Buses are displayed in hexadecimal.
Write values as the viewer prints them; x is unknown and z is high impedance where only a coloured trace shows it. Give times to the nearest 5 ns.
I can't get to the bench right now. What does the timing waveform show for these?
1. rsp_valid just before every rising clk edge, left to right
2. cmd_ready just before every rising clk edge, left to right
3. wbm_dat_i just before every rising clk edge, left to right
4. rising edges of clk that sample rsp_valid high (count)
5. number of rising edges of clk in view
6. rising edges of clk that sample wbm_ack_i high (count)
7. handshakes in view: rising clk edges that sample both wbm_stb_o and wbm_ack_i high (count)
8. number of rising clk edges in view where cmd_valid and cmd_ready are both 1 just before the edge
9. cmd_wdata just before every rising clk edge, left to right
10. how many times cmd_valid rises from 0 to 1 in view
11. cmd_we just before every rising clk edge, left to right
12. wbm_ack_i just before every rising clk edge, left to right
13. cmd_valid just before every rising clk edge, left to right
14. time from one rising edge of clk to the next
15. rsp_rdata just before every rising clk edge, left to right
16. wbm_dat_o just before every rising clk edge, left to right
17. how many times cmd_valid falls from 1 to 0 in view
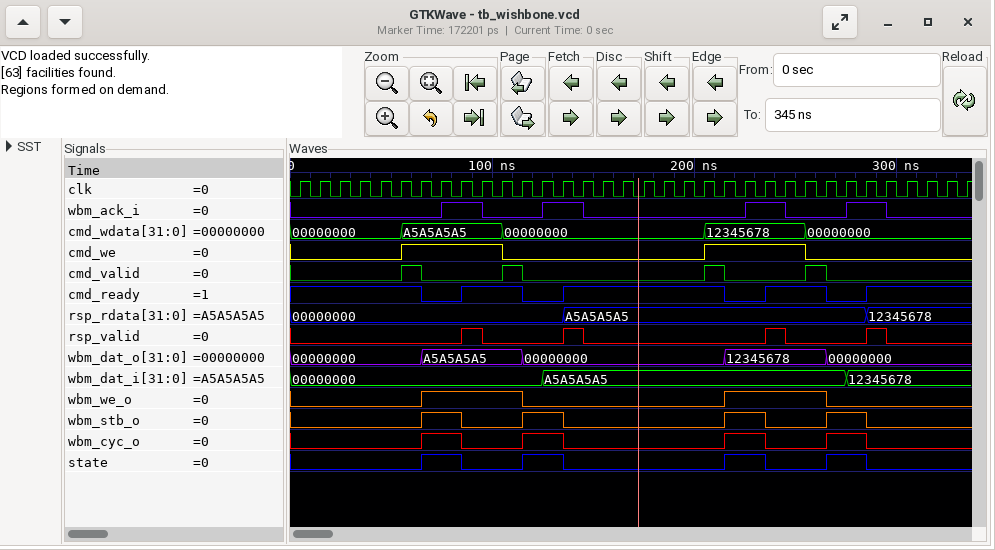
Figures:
0 0 0 0 0 0 0 0 0 1 0 0 0 0 1 0 0 0 0 0 0 0 0 0 1 0 0 0 0 1 0 0 0 0
1 1 1 1 1 1 1 0 0 1 1 1 0 0 1 1 1 1 1 1 1 1 0 0 1 1 1 0 0 1 1 1 1 1
00000000, 00000000, 00000000, 00000000, 00000000, 00000000, 00000000, 00000000, 00000000, 00000000, 00000000, 00000000, 00000000, A5A5A5A5, A5A5A5A5, A5A5A5A5, A5A5A5A5, A5A5A5A5, A5A5A5A5, A5A5A5A5, A5A5A5A5, A5A5A5A5, A5A5A5A5, A5A5A5A5, A5A5A5A5, A5A5A5A5, A5A5A5A5, A5A5A5A5, 12345678, 12345678, 12345678, 12345678, 12345678, 12345678
4
34
8
4
4
00000000, 00000000, 00000000, 00000000, 00000000, 00000000, A5A5A5A5, A5A5A5A5, A5A5A5A5, A5A5A5A5, A5A5A5A5, 00000000, 00000000, 00000000, 00000000, 00000000, 00000000, 00000000, 00000000, 00000000, 00000000, 12345678, 12345678, 12345678, 12345678, 12345678, 00000000, 00000000, 00000000, 00000000, 00000000, 00000000, 00000000, 00000000
4
0 0 0 0 0 0 1 1 1 1 1 0 0 0 0 0 0 0 0 0 0 1 1 1 1 1 0 0 0 0 0 0 0 0
0 0 0 0 0 0 0 0 1 1 0 0 0 1 1 0 0 0 0 0 0 0 0 1 1 0 0 0 1 1 0 0 0 0
0 0 0 0 0 0 1 0 0 0 0 1 0 0 0 0 0 0 0 0 0 1 0 0 0 0 1 0 0 0 0 0 0 0
10 ns
00000000, 00000000, 00000000, 00000000, 00000000, 00000000, 00000000, 00000000, 00000000, 00000000, 00000000, 00000000, 00000000, 00000000, A5A5A5A5, A5A5A5A5, A5A5A5A5, A5A5A5A5, A5A5A5A5, A5A5A5A5, A5A5A5A5, A5A5A5A5, A5A5A5A5, A5A5A5A5, A5A5A5A5, A5A5A5A5, A5A5A5A5, A5A5A5A5, A5A5A5A5, 12345678, 12345678, 12345678, 12345678, 12345678
00000000, 00000000, 00000000, 00000000, 00000000, 00000000, 00000000, A5A5A5A5, A5A5A5A5, A5A5A5A5, A5A5A5A5, A5A5A5A5, 00000000, 00000000, 00000000, 00000000, 00000000, 00000000, 00000000, 00000000, 00000000, 00000000, 12345678, 12345678, 12345678, 12345678, 12345678, 00000000, 00000000, 00000000, 00000000, 00000000, 00000000, 00000000
4
